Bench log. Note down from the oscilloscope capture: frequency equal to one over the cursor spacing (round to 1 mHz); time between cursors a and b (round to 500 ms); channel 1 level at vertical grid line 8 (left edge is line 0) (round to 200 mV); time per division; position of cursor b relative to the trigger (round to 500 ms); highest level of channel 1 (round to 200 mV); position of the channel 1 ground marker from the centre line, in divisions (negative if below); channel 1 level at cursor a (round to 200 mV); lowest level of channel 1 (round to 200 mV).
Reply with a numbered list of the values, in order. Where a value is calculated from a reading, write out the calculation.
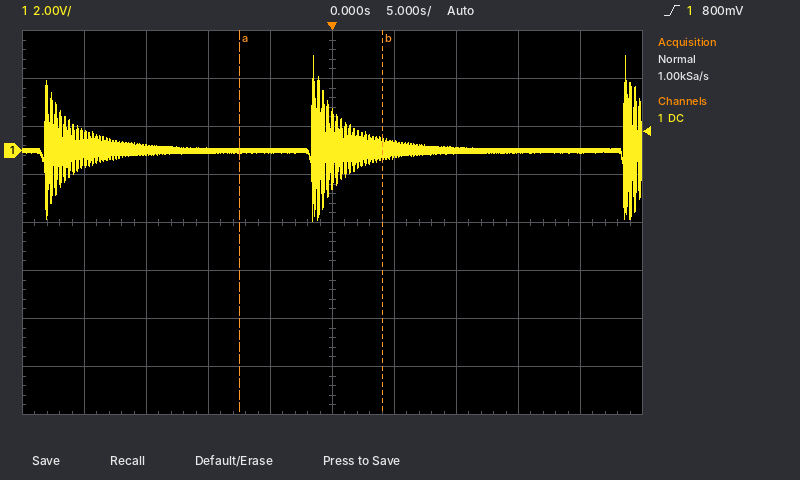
1. 1 / 11.5 s ≈ 87 mHz
2. 11.5 s
3. 0.0 V
4. 5 s
5. +4.0 s
6. 4.0 V
7. +1.5 div
8. 0.0 V
9. -3.0 V
